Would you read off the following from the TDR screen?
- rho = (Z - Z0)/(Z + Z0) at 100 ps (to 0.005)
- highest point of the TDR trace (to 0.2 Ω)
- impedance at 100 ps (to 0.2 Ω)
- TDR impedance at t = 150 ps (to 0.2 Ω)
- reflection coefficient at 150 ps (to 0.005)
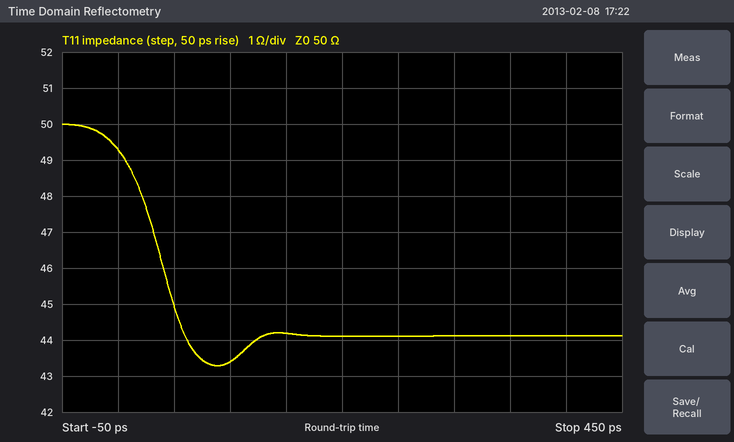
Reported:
-0.070
50.0 Ω
43.4 Ω
44.2 Ω
-0.060
